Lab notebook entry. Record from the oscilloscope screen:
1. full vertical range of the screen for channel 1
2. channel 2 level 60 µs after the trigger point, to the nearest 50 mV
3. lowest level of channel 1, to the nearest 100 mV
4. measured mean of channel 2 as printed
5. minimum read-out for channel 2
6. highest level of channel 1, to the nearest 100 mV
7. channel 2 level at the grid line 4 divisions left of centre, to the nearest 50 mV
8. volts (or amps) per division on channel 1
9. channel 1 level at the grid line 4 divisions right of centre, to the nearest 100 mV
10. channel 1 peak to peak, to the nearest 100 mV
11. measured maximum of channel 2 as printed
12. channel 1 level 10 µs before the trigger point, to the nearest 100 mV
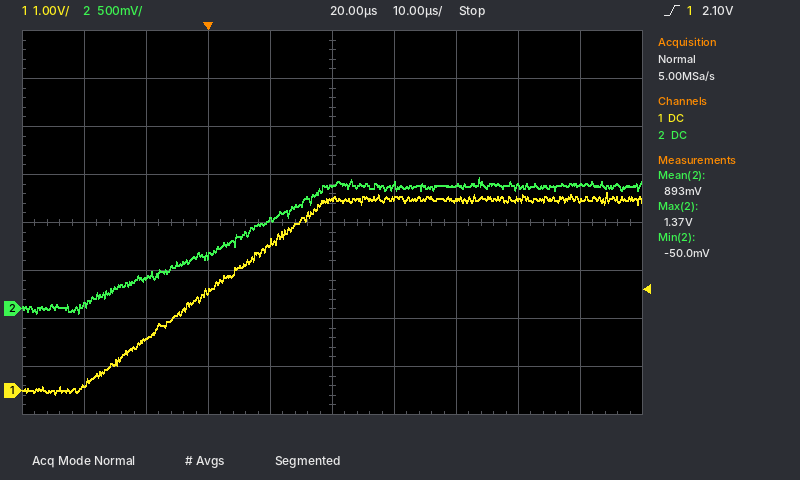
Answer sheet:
8 V
1.30 V
-100 mV
893 mV
-50.0 mV
4.1 V
50 mV
1 V
4.0 V
4.2 V
1.37 V
1.1 V
